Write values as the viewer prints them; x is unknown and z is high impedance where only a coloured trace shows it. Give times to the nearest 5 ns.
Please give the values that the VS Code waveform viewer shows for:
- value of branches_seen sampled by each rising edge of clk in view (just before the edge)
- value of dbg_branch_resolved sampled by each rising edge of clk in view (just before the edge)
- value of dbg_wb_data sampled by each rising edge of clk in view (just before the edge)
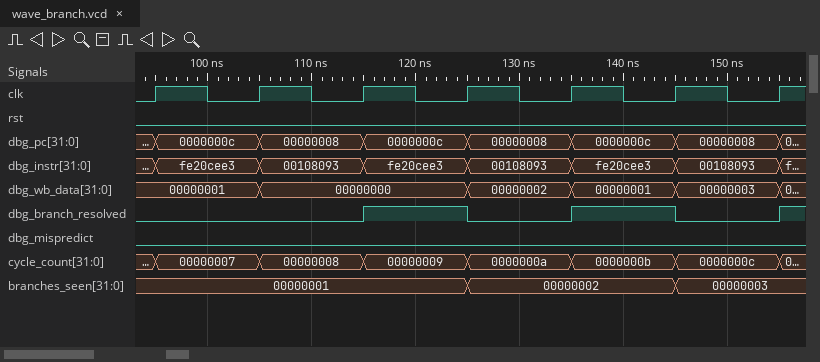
00000001, 00000001, 00000001, 00000001, 00000002, 00000002, 00000003
0 0 0 1 0 1 0
00000001, 00000001, 00000000, 00000000, 00000002, 00000001, 00000003
